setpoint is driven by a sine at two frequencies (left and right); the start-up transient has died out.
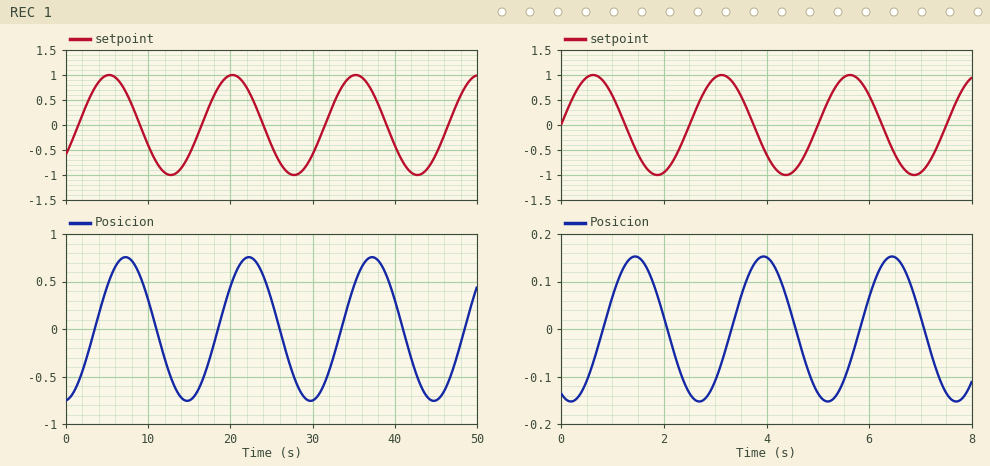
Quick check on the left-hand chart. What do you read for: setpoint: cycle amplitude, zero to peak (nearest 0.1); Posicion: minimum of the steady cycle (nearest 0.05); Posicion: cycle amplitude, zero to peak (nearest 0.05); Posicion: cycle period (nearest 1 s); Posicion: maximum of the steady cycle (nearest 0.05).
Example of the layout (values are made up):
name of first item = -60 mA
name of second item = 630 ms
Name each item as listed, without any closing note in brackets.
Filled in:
setpoint: cycle amplitude, zero to peak = 1.0
Posicion: minimum of the steady cycle = -0.75
Posicion: cycle amplitude, zero to peak = 0.75
Posicion: cycle period = 15 s
Posicion: maximum of the steady cycle = 0.75
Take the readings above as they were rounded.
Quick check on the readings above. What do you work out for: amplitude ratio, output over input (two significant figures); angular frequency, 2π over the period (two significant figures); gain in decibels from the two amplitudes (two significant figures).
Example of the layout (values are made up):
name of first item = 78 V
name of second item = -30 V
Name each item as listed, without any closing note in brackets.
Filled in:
amplitude ratio, output over input = 0.75
angular frequency, 2π over the period = 0.42 rad/s
gain in decibels from the two amplitudes = -2.5 dB
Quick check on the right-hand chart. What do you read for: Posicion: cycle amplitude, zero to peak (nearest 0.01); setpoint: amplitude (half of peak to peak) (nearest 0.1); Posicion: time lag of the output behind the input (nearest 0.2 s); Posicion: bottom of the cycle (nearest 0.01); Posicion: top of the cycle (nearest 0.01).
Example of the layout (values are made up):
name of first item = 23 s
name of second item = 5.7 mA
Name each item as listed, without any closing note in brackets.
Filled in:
Posicion: cycle amplitude, zero to peak = 0.15
setpoint: amplitude (half of peak to peak) = 1.0
Posicion: time lag of the output behind the input = 0.8 s
Posicion: bottom of the cycle = -0.15
Posicion: top of the cycle = 0.15
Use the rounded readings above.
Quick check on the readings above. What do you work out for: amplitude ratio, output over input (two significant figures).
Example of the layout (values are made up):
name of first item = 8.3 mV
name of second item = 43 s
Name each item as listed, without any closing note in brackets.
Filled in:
amplitude ratio, output over input = 0.15
